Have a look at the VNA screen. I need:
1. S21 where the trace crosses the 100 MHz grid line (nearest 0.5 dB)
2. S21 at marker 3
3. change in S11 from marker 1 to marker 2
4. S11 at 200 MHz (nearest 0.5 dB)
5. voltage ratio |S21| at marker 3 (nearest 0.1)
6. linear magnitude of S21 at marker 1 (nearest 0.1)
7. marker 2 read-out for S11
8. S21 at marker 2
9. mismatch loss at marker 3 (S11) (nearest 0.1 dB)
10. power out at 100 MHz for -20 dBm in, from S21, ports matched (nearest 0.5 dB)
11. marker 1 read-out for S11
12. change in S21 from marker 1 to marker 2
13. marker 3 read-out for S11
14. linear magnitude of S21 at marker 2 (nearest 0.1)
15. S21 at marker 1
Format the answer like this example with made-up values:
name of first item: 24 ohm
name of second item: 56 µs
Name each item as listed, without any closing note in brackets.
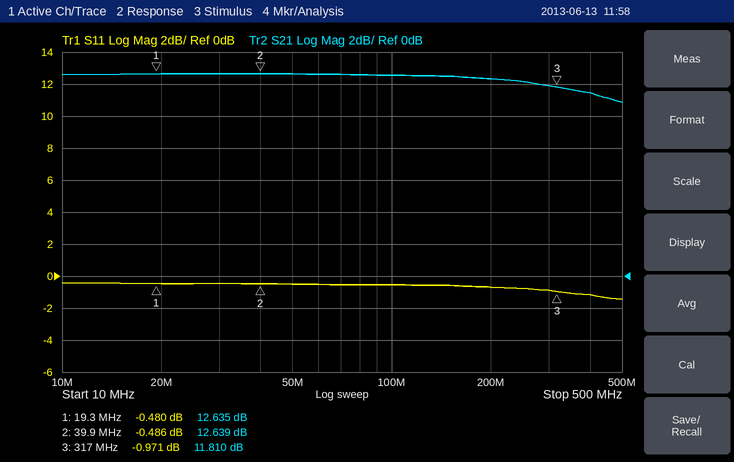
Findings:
S21 where the trace crosses the 100 MHz grid line: 12.5 dB
S21 at marker 3: 11.810 dB
change in S11 from marker 1 to marker 2: -0.006 dB
S11 at 200 MHz: -0.5 dB
voltage ratio |S21| at marker 3: 3.9
linear magnitude of S21 at marker 1: 4.3
marker 2 read-out for S11: -0.486 dB
S21 at marker 2: 12.639 dB
mismatch loss at marker 3 (S11): 7.0 dB
power out at 100 MHz for -20 dBm in, from S21, ports matched: -7.5 dBm
marker 1 read-out for S11: -0.480 dB
change in S21 from marker 1 to marker 2: 0.004 dB
marker 3 read-out for S11: -0.971 dB
linear magnitude of S21 at marker 2: 4.3
S21 at marker 1: 12.635 dB
